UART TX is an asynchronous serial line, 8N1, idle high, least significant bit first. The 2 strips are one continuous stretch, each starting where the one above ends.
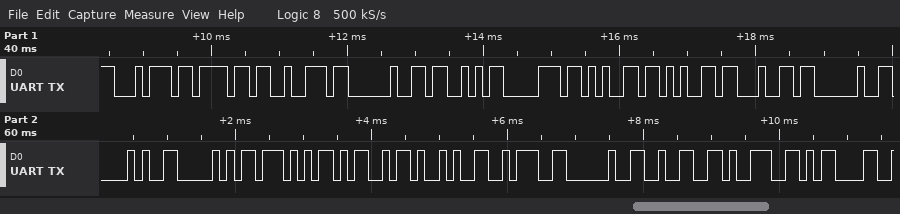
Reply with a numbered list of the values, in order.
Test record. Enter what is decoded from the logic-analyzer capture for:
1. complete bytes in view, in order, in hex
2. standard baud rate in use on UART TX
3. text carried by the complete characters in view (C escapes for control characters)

1. 0x74 0x6F 0x72 0x20 0x53 0x70 0x65 0x65 0x64 0x20 0x28 0x50 0x57 0x4D 0x29 0x3A 0x20 0x32 0x39 0x0D
2. 9600 baud
3. "tor Speed (PWM): 29\r"
